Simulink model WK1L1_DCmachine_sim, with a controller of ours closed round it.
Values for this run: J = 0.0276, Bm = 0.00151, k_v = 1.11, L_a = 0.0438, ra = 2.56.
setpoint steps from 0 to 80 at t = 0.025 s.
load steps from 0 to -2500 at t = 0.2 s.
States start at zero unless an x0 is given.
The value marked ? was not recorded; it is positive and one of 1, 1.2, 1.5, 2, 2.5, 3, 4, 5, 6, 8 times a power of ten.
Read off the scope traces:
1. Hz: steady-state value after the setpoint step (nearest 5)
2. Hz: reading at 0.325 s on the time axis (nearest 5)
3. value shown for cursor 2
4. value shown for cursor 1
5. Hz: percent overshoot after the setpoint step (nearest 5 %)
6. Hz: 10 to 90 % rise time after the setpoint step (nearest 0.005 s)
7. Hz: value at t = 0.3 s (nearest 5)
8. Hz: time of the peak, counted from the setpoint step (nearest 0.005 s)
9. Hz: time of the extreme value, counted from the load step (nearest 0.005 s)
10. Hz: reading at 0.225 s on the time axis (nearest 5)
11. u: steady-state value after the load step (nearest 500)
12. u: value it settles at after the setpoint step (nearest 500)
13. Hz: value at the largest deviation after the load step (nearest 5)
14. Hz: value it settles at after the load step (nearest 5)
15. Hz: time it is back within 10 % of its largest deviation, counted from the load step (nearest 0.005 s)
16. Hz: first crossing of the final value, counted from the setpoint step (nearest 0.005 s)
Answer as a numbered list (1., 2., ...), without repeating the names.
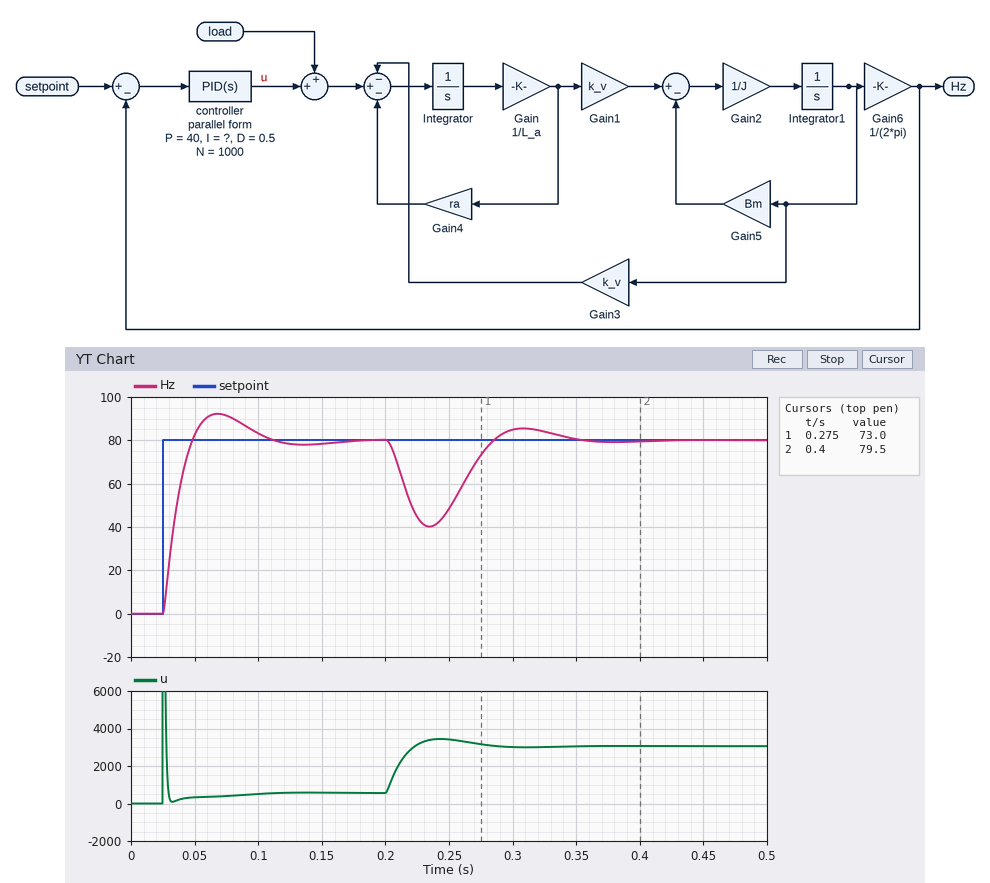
1. 80
2. 85
3. 79.5
4. 73.0
5. 15 %
6. 0.015 s
7. 85
8. 0.045 s
9. 0.035 s
10. 45
11. 3000
12. 500
13. 40
14. 80
15. 0.125 s
16. 0.025 s
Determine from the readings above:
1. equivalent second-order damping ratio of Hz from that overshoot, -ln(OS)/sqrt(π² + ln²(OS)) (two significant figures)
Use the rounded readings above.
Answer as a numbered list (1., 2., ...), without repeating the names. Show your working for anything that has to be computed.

1. ln(0.15) = -1.897; 1.897 / sqrt(9.870 + 3.599) = 0.52
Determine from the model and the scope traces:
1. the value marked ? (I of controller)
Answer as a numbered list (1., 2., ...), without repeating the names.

1. 1500
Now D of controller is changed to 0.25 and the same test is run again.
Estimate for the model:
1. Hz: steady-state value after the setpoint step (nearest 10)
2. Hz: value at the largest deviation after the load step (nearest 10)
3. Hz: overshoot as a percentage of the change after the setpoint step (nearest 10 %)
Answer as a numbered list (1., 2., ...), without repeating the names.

1. 80
2. 30
3. 30 %
